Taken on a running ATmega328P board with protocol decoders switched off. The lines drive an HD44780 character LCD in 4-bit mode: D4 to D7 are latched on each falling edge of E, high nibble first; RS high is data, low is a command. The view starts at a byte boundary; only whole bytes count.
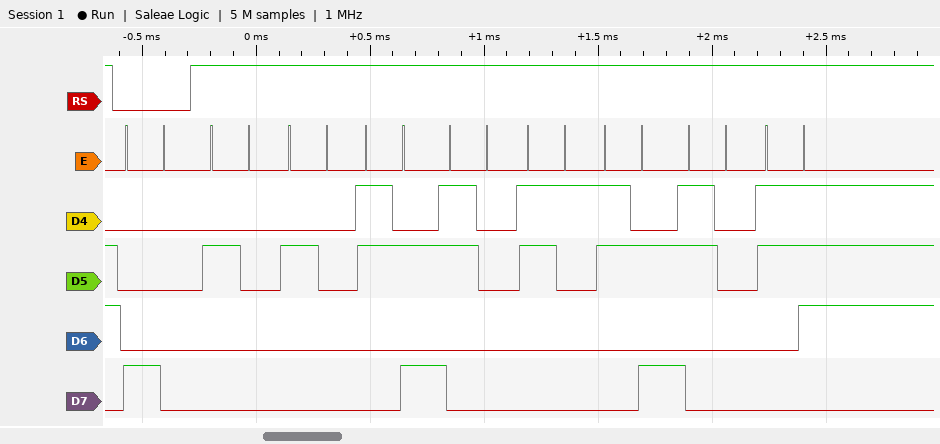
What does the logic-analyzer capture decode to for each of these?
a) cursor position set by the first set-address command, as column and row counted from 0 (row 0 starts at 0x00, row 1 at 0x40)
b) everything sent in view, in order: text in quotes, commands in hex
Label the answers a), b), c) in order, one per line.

a) column 0, row 0
b) 0x80 "  :01:07"
